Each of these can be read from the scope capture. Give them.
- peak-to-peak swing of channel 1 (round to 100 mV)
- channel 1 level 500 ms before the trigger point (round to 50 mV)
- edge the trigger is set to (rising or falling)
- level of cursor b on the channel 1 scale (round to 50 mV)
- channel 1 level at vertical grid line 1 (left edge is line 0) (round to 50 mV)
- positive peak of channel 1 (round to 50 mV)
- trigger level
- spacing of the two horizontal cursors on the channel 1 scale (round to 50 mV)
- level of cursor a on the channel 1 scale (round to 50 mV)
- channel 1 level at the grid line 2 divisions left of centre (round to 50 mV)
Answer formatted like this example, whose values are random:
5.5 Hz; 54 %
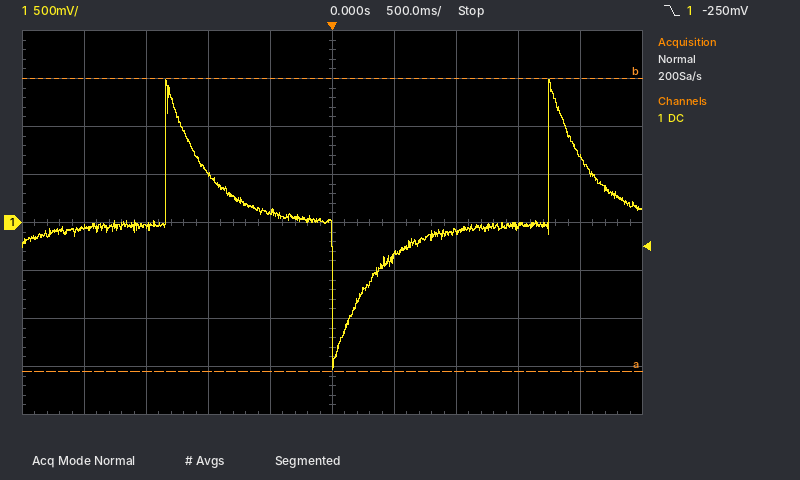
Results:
3.00 V; 100 mV; falling; 1.50 V; -50 mV; 1.50 V; -250 mV; 3.05 V; -1.55 V; 500 mV
